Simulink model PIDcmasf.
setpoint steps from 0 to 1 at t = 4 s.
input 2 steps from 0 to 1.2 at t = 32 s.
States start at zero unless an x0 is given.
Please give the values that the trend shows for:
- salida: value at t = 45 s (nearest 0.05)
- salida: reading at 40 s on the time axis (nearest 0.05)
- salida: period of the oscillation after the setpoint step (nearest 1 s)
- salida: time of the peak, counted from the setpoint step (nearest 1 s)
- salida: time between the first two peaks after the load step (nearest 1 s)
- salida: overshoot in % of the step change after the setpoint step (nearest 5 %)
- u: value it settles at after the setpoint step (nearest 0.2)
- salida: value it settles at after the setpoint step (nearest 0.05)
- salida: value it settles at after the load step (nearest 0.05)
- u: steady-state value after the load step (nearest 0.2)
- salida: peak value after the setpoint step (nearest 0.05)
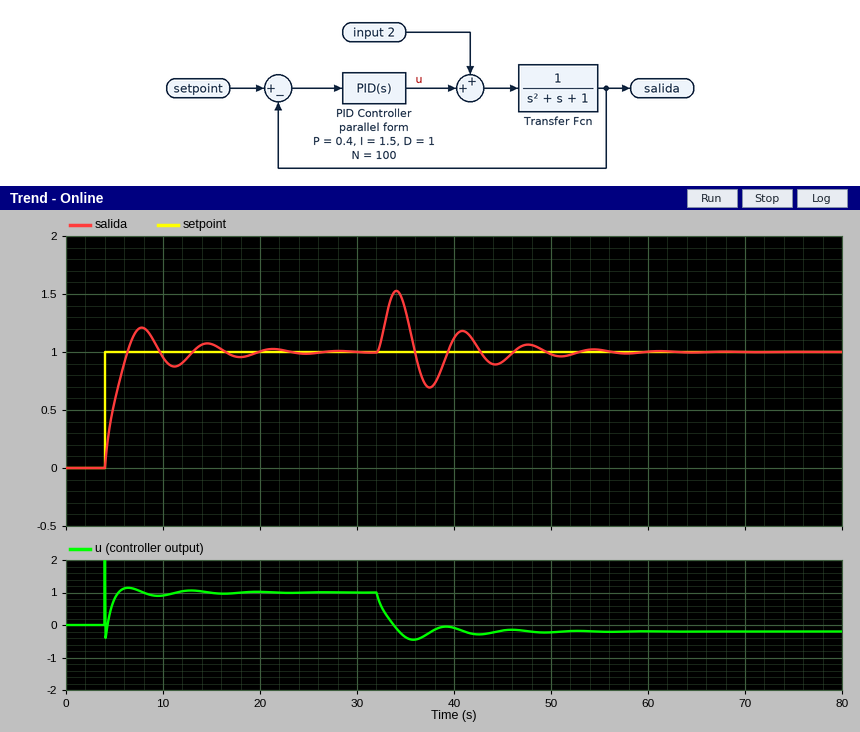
0.90
1.10
7 s
4 s
7 s
20 %
1.0
1.00
1.00
-0.2
1.20
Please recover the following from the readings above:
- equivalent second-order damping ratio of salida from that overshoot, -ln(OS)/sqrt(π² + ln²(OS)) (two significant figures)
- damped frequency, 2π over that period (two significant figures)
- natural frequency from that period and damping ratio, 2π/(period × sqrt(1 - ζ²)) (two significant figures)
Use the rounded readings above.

0.46
0.90 rad/s
1.0 rad/s
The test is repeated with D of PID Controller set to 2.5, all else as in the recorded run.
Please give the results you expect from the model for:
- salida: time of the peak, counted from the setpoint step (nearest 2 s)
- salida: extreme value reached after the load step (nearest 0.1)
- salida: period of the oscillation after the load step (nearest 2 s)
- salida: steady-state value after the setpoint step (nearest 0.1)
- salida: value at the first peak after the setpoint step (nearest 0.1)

6 s
1.4
10 s
1.0
1.1
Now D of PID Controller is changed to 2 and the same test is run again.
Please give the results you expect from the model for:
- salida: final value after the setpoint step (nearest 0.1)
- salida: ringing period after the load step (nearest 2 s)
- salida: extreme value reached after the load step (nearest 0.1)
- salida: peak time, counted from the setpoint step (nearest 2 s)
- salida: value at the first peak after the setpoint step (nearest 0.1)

1.0
8 s
1.4
6 s
1.1
